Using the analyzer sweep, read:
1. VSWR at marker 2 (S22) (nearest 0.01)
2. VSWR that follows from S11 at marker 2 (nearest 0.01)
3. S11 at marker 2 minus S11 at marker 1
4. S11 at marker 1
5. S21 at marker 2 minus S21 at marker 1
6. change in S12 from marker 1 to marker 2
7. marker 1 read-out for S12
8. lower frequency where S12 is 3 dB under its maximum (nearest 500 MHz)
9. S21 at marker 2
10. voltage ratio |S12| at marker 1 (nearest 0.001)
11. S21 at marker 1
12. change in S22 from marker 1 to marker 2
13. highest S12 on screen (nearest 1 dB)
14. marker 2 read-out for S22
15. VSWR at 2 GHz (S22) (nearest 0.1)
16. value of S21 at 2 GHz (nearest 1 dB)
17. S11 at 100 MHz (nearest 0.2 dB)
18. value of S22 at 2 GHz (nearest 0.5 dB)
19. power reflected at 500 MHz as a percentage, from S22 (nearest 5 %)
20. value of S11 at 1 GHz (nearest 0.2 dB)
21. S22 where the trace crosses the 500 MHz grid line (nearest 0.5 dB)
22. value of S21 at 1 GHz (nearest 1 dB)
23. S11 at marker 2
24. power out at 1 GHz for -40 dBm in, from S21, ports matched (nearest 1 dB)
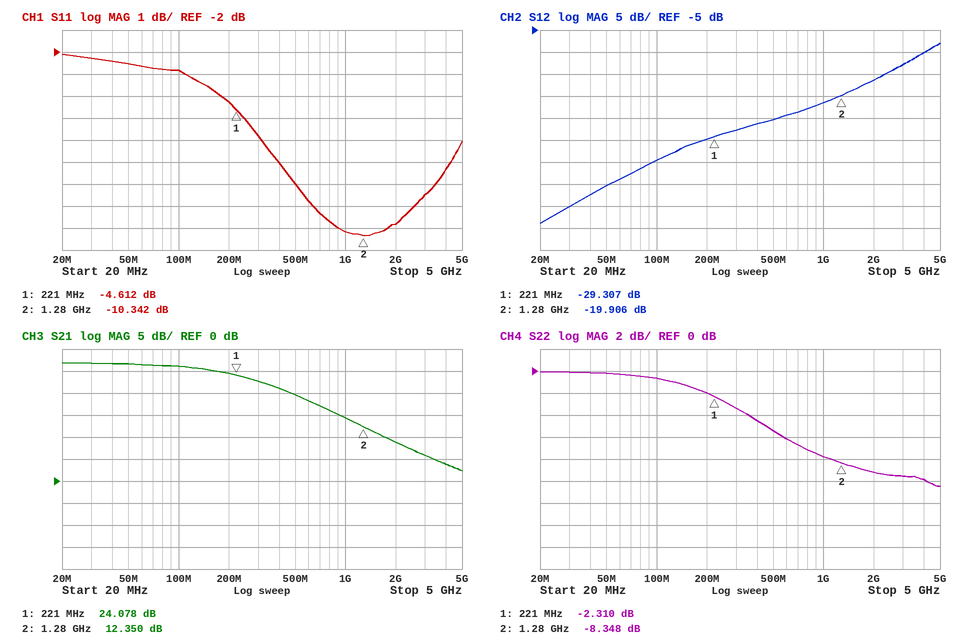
2.24
1.87
-5.730 dB
-4.612 dB
-11.728 dB
9.401 dB
-29.307 dB
3.5 GHz
12.350 dB
0.034
24.078 dB
-6.038 dB
-8 dB
-8.348 dB
2.1
9 dB
-2.8 dB
-9.0 dB
30 %
-10.2 dB
-5.5 dB
14 dB
-10.342 dB
-26 dBm
